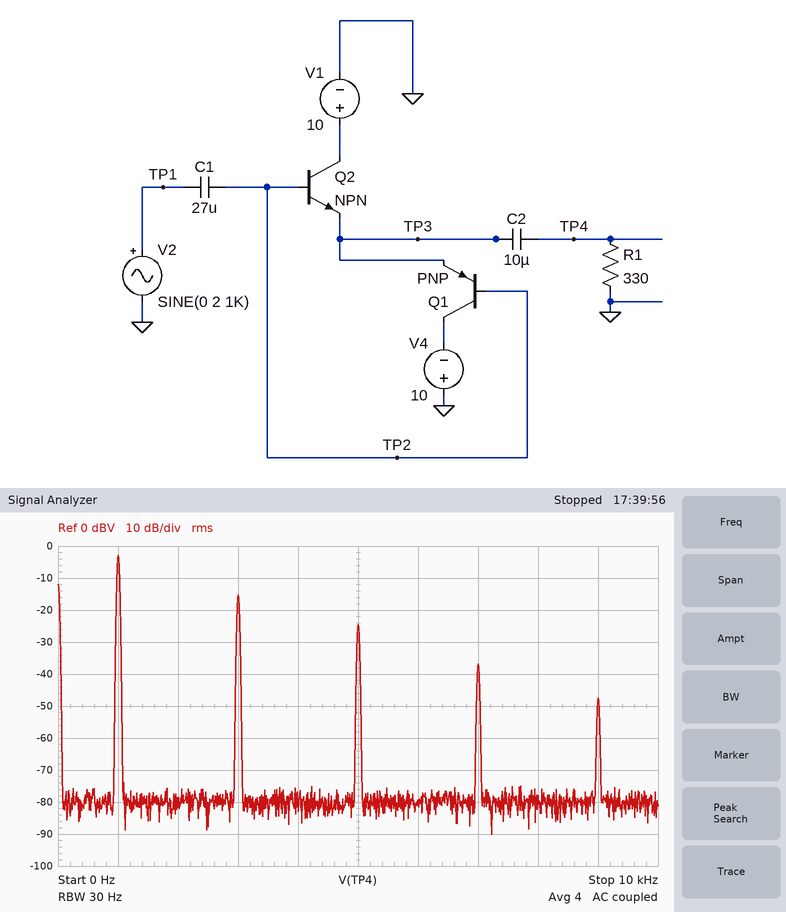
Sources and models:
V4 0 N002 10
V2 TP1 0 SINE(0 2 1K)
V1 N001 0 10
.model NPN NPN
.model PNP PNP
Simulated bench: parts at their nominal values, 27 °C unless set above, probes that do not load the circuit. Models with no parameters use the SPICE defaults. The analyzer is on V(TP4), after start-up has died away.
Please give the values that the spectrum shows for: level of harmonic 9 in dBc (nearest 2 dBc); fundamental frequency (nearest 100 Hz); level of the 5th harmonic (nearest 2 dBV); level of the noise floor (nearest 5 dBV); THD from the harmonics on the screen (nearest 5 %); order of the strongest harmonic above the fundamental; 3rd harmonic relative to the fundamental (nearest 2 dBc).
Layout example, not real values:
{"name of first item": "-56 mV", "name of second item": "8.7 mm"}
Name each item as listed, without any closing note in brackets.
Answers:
{"level of harmonic 9 in dBc": "-44 dBc", "fundamental frequency": "1.0 kHz", "level of the 5th harmonic": "-24 dBV", "level of the noise floor": "-80 dBV", "THD from the harmonics on the screen": "25 %", "order of the strongest harmonic above the fundamental": "3", "3rd harmonic relative to the fundamental": "-12 dBc"}
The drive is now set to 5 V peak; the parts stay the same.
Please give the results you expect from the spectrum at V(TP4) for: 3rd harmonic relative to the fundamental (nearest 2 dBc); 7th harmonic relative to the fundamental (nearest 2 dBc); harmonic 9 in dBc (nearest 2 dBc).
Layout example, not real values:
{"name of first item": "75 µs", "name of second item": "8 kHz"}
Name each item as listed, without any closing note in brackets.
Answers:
{"3rd harmonic relative to the fundamental": "-22 dBc", "7th harmonic relative to the fundamental": "-32 dBc", "harmonic 9 in dBc": "-34 dBc"}
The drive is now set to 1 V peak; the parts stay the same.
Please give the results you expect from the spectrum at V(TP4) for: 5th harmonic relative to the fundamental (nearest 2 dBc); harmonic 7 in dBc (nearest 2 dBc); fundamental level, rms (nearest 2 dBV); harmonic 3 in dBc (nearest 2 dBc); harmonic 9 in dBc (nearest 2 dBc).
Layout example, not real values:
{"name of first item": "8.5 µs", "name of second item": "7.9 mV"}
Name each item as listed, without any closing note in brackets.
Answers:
{"5th harmonic relative to the fundamental": "-18 dBc", "harmonic 7 in dBc": "-24 dBc", "fundamental level, rms": "-20 dBV", "harmonic 3 in dBc": "-4 dBc", "harmonic 9 in dBc": "-30 dBc"}
